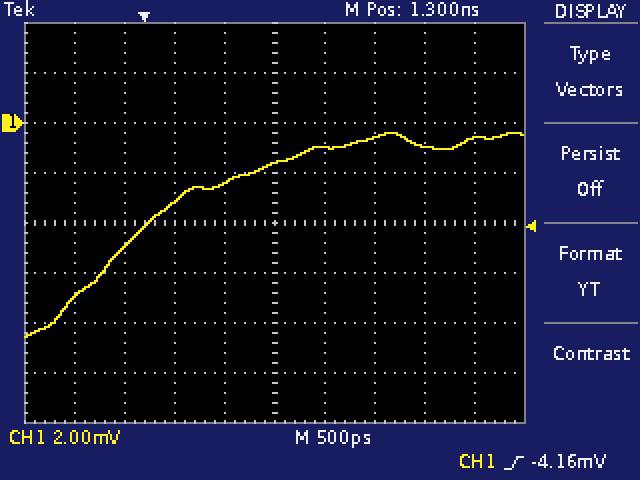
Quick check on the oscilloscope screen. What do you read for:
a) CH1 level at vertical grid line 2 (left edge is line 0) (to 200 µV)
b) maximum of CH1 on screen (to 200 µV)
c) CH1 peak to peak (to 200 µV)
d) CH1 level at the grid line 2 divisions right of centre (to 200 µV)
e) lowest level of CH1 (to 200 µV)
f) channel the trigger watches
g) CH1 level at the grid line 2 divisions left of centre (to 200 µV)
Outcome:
-5.0 mV
-400 µV
8.2 mV
-600 µV
-8.6 mV
CH1
-3.2 mV
